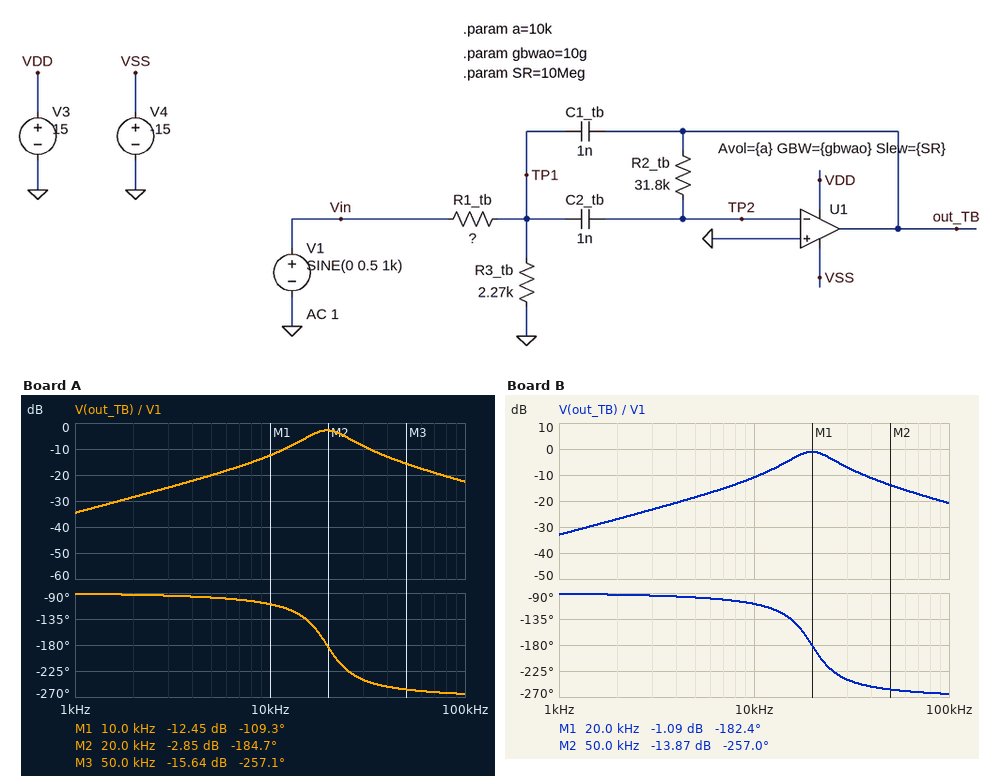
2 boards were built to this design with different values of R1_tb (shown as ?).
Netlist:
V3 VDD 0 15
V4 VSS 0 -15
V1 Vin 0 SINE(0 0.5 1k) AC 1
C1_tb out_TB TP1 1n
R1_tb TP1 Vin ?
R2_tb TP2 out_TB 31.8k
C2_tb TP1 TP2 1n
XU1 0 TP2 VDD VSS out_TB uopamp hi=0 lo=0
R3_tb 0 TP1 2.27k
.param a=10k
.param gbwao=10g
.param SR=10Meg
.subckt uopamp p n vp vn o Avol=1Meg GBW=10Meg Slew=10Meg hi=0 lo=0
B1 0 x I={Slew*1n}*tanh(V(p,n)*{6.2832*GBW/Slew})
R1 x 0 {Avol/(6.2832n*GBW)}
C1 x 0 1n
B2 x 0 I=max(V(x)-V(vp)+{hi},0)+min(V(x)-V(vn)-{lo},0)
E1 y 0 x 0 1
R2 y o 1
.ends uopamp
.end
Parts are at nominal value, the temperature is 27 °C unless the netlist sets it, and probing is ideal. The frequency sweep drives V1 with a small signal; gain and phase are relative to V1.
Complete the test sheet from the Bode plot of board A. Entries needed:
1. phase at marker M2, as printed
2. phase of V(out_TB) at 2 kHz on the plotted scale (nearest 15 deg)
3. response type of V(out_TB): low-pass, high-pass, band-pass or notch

-184.7 deg
-90 deg
band-pass
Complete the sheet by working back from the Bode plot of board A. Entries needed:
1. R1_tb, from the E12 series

22 kΩ
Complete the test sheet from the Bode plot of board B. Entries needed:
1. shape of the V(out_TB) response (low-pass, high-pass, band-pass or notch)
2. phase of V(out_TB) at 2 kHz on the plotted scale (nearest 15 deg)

band-pass
-90 deg
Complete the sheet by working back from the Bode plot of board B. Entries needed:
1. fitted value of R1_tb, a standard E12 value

18 kΩ
